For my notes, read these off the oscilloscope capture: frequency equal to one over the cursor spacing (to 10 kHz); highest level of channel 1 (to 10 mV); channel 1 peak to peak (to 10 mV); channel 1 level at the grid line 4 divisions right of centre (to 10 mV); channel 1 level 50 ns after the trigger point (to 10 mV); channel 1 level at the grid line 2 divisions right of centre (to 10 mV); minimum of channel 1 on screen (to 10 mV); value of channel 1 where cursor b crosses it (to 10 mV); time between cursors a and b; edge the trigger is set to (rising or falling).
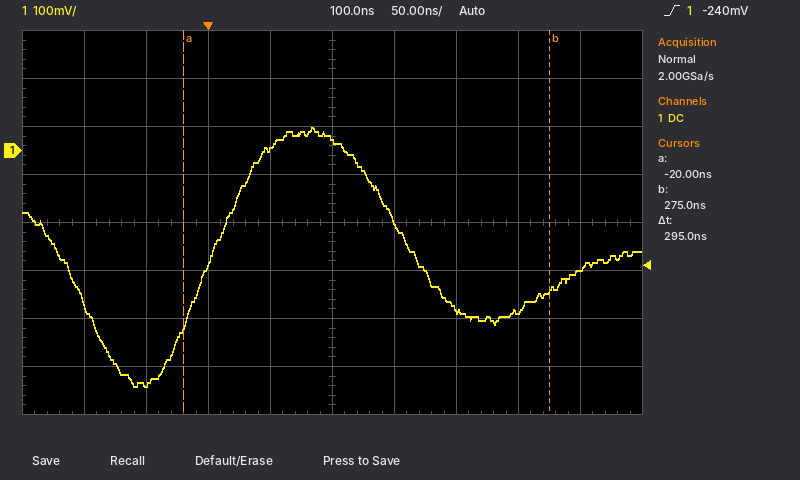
3.39 MHz
50 mV
540 mV
-250 mV
0 mV
-330 mV
-490 mV
-290 mV
295 ns
rising
